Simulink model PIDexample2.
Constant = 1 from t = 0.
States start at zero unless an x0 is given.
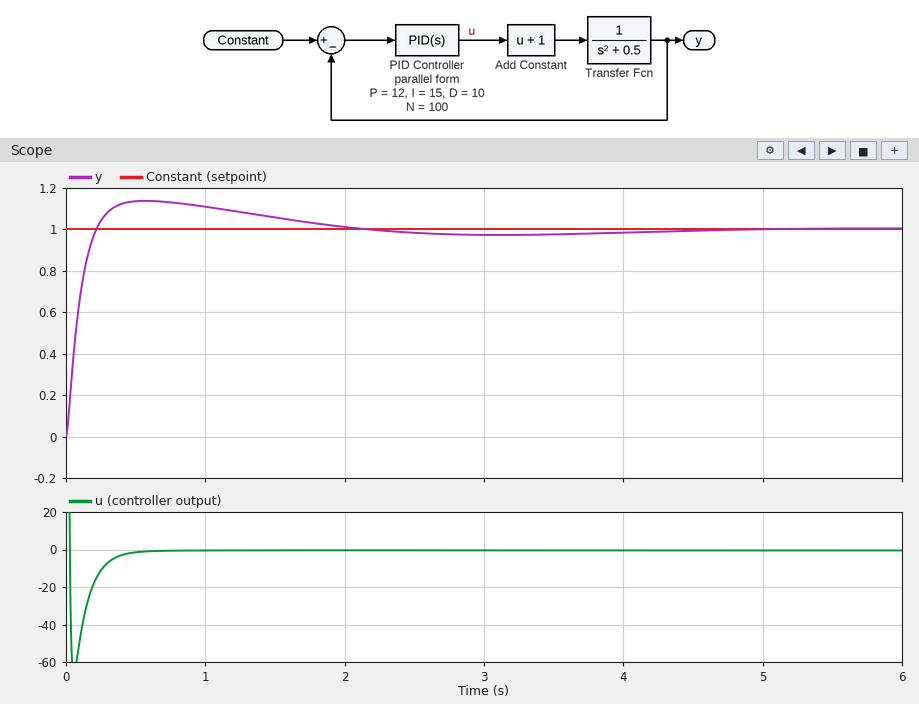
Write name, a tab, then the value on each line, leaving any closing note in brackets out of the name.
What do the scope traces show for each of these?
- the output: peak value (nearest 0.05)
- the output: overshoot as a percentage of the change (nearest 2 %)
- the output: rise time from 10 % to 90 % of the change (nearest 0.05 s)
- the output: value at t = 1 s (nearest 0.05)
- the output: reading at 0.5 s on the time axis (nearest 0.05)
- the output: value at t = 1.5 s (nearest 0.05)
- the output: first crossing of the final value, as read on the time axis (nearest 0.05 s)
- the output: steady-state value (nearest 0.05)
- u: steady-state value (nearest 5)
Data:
the output: peak value	1.15
the output: overshoot as a percentage of the change	14 %
the output: rise time from 10 % to 90 % of the change	0.15 s
the output: value at t = 1 s	1.10
the output: reading at 0.5 s on the time axis	1.15
the output: value at t = 1.5 s	1.05
the output: first crossing of the final value, as read on the time axis	0.20 s
the output: steady-state value	1.00
u: steady-state value	0
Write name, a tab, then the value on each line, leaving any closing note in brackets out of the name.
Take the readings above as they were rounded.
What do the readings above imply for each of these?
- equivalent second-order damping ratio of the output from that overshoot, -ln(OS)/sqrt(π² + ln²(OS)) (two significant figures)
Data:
equivalent second-order damping ratio of the output from that overshoot, -ln(OS)/sqrt(π² + ln²(OS))	0.53
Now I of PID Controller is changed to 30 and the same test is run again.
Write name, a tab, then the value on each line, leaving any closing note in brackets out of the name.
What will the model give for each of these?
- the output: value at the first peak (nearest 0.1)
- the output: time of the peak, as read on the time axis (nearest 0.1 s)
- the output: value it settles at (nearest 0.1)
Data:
the output: value at the first peak	1.2
the output: time of the peak, as read on the time axis	0.6 s
the output: value it settles at	1.0
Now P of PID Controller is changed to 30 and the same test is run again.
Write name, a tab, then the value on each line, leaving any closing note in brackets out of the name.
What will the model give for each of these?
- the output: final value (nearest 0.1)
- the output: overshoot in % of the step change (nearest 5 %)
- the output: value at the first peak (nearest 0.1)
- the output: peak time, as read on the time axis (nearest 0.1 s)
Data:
the output: final value	1.0
the output: overshoot in % of the step change	20 %
the output: value at the first peak	1.2
the output: peak time, as read on the time axis	0.4 s
